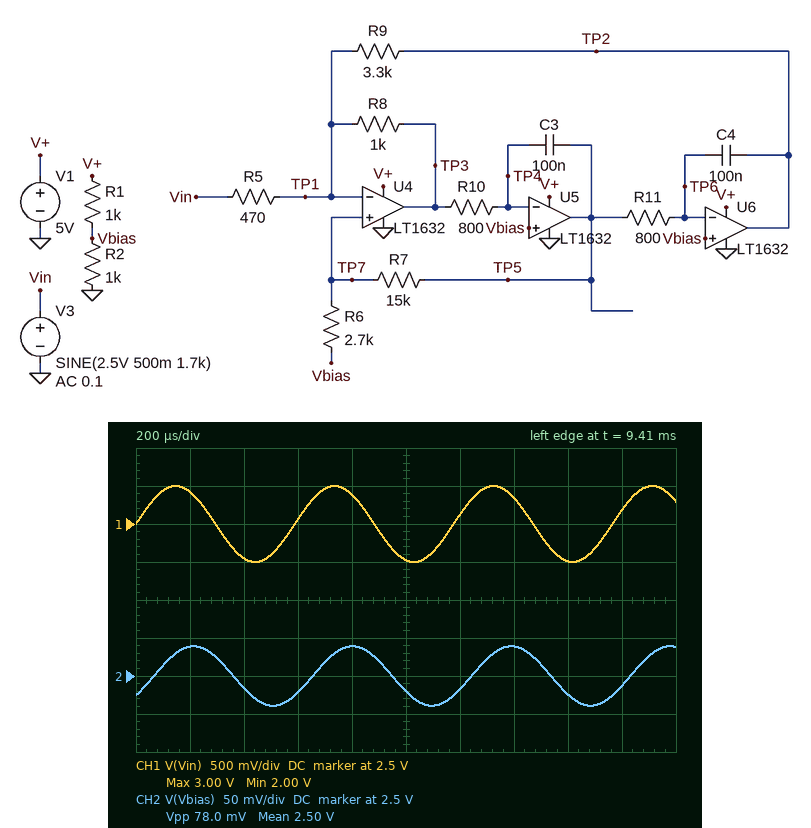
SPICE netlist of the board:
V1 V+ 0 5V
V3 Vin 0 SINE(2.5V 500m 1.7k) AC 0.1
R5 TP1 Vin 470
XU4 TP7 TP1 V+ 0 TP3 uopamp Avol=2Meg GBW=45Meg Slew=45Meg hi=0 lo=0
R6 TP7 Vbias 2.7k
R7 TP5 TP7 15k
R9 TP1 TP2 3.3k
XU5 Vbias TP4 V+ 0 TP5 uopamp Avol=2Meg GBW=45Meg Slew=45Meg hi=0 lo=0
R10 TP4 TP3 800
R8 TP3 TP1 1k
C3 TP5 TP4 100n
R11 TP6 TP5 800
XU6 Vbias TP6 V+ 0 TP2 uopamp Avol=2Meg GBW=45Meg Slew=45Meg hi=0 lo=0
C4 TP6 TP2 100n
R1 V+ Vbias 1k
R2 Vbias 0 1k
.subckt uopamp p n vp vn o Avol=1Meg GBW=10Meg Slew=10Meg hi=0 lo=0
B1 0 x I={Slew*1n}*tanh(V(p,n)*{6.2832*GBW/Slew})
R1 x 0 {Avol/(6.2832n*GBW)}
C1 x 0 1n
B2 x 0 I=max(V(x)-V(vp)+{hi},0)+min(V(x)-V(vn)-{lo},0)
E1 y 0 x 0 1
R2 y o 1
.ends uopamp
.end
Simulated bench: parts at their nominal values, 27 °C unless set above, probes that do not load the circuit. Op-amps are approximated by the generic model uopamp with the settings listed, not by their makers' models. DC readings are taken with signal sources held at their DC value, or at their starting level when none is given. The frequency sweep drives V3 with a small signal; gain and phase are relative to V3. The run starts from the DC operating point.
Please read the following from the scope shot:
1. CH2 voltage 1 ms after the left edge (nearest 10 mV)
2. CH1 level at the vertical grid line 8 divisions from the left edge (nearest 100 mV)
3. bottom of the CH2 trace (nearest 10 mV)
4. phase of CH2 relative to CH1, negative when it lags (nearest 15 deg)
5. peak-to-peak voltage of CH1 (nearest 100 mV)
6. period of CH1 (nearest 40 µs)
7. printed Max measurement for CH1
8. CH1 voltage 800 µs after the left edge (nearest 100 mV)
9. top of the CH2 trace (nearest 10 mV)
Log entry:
2.48 V
2.0 V
2.46 V
-45 deg
1.0 V
600 µs
3.00 V
2.9 V
2.54 V
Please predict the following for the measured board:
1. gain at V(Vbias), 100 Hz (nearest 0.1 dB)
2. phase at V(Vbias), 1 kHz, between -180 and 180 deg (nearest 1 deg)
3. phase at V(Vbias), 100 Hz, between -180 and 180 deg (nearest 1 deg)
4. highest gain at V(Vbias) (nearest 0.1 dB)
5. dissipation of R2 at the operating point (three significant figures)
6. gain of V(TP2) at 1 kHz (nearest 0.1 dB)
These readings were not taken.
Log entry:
-40.0 dB
10 deg
84 deg
-19.7 dB
6.25 mW
17.1 dB
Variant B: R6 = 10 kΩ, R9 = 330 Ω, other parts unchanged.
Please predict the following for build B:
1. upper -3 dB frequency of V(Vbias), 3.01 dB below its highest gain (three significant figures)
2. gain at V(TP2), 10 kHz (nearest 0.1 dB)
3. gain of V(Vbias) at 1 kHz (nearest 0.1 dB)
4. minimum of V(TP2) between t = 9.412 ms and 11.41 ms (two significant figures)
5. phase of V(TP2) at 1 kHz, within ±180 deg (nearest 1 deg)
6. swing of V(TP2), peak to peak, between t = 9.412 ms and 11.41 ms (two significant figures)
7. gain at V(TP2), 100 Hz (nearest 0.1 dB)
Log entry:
6.76 kHz
-21.5 dB
-43.1 dB
2.2 V
155 deg
680 mV
-3.1 dB
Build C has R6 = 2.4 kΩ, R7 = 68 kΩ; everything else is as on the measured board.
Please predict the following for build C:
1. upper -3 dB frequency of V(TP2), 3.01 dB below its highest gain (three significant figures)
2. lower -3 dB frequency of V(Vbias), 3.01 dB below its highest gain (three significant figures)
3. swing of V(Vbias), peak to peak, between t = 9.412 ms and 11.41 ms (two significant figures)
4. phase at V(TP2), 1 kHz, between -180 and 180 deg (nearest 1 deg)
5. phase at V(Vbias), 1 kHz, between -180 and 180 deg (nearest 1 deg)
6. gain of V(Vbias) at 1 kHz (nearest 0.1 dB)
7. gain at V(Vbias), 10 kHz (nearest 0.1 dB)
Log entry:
1.20 kHz
972 Hz
29 mV
127 deg
37 deg
-20.8 dB
-50.3 dB
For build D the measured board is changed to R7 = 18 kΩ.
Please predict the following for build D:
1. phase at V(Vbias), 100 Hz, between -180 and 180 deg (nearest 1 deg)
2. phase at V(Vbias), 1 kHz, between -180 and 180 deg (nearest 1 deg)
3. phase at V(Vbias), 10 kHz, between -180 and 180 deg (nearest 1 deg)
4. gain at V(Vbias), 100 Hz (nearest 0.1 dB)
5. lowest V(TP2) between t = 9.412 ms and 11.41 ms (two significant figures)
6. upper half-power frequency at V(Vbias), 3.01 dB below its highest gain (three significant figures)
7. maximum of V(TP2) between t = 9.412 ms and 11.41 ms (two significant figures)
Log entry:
85 deg
11 deg
-84 deg
-41.3 dB
740 mV
1.70 kHz
4.3 V
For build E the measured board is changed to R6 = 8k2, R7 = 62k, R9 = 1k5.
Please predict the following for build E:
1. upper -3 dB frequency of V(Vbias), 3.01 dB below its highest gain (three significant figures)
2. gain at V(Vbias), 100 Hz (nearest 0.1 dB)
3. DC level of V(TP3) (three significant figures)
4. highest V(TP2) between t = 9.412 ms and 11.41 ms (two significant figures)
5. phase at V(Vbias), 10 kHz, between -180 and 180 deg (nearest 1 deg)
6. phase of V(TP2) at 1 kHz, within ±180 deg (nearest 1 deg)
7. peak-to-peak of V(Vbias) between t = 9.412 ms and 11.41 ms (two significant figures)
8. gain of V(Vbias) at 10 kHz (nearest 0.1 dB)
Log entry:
2.14 kHz
-58.8 dB
2.50 V
5.0 V
-85 deg
151 deg
32 mV
-50.2 dB
